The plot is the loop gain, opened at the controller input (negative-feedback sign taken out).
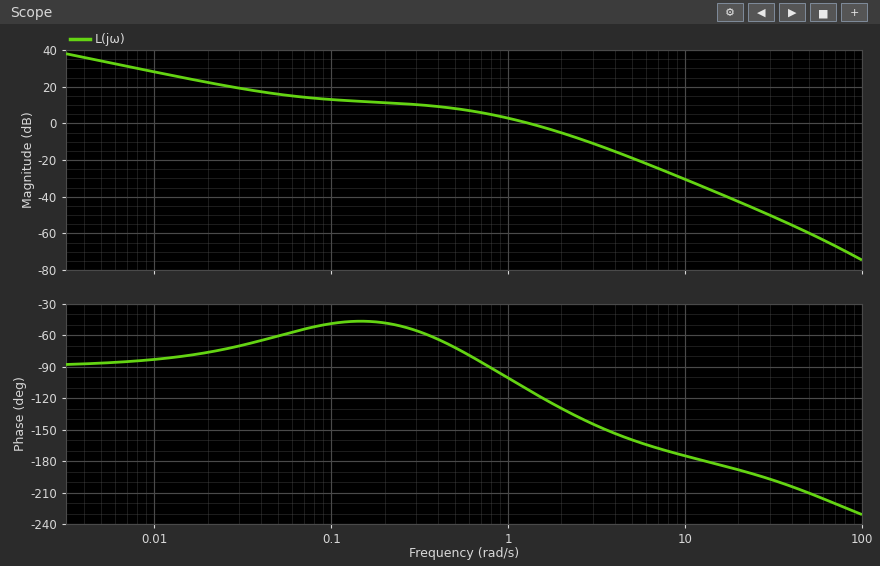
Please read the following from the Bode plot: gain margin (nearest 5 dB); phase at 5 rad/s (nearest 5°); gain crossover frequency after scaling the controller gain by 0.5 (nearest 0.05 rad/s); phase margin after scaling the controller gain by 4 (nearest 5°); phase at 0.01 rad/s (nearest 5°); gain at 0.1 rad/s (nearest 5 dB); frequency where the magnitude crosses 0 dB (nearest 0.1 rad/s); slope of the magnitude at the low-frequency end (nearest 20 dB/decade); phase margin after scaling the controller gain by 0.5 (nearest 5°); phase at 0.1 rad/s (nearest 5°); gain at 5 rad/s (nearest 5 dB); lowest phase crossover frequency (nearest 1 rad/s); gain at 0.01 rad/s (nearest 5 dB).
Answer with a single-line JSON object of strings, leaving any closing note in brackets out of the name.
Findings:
{"gain margin": "35 dB", "phase at 5 rad/s": "-160°", "gain crossover frequency after scaling the controller gain by 0.5": "0.70 rad/s", "phase margin after scaling the controller gain by 4": "35°", "phase at 0.01 rad/s": "-85°", "gain at 0.1 rad/s": "15 dB", "frequency where the magnitude crosses 0 dB": "1.3 rad/s", "slope of the magnitude at the low-frequency end": "-20 dB/decade", "phase margin after scaling the controller gain by 0.5": "95°", "phase at 0.1 rad/s": "-50°", "gain at 5 rad/s": "-20 dB", "lowest phase crossover frequency": "13 rad/s", "gain at 0.01 rad/s": "30 dB"}
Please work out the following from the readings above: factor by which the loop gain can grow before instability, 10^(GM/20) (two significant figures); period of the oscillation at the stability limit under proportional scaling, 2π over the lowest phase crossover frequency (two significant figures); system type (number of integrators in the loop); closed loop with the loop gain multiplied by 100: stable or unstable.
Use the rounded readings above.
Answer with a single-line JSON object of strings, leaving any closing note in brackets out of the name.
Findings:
{"factor by which the loop gain can grow before instability, 10^(GM/20)": "56", "period of the oscillation at the stability limit under proportional scaling, 2π over the lowest phase crossover frequency": "0.48 s", "system type": "1", "closed loop with the loop gain multiplied by 100: stable or unstable": "unstable"}
